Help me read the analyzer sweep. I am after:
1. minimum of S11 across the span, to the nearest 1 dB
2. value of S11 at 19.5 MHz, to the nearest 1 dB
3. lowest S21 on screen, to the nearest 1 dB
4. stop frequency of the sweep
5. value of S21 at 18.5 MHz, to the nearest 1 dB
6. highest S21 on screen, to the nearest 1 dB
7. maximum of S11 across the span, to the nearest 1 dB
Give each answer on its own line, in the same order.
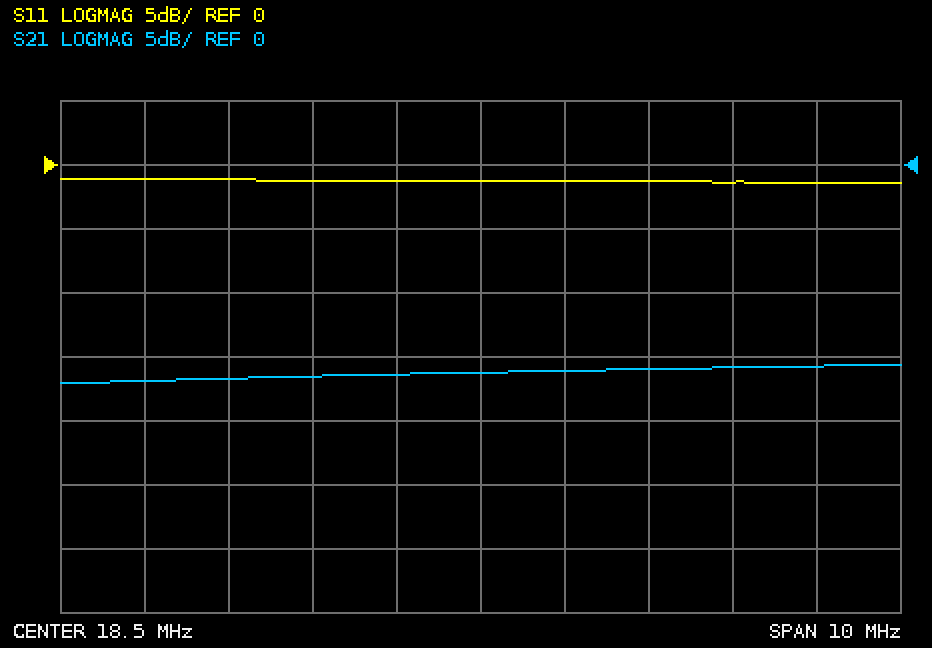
-1 dB
-1 dB
-17 dB
23.5 MHz
-16 dB
-16 dB
-1 dB
